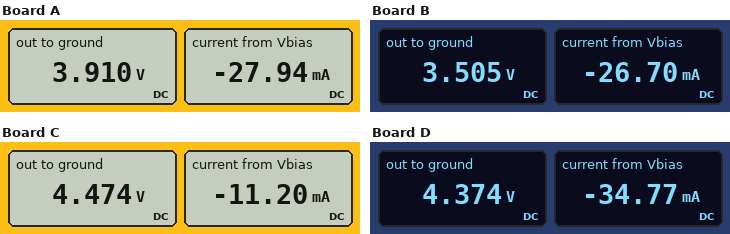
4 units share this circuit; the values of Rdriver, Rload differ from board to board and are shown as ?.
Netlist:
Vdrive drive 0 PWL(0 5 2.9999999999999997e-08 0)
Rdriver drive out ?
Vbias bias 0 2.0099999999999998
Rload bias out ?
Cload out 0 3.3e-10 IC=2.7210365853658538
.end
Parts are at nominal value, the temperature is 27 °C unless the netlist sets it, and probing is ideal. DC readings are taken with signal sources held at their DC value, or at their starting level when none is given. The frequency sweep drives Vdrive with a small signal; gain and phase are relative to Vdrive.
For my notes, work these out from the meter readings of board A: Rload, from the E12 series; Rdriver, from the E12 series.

68 Ω
39 Ω
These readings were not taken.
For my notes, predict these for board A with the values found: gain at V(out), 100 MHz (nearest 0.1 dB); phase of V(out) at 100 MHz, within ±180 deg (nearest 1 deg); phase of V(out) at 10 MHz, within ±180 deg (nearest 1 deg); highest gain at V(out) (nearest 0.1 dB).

-18.3 dB
-79 deg
-27 deg
-3.9 dB
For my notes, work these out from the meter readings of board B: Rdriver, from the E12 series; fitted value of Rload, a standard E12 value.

56 Ω
56 Ω
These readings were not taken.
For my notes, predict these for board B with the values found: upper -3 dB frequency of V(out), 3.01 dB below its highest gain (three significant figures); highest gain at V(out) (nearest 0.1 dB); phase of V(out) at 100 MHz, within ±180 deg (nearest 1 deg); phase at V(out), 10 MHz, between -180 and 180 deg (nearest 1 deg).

17.2 MHz
-6.0 dB
-80 deg
-30 deg
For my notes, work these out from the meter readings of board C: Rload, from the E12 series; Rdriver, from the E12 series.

220 Ω
47 Ω
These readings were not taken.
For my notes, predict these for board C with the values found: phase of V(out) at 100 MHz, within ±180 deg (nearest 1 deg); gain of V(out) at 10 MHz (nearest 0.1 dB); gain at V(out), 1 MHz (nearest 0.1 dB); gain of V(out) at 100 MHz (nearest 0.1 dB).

-83 deg
-3.8 dB
-1.7 dB
-19.8 dB
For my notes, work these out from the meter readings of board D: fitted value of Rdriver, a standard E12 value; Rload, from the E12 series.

18 Ω
68 Ω
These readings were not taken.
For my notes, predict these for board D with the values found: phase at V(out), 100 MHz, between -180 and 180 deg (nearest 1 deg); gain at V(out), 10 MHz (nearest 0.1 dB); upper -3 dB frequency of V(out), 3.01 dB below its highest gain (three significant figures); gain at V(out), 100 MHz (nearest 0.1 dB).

-71 deg
-2.4 dB
33.9 MHz
-11.9 dB
